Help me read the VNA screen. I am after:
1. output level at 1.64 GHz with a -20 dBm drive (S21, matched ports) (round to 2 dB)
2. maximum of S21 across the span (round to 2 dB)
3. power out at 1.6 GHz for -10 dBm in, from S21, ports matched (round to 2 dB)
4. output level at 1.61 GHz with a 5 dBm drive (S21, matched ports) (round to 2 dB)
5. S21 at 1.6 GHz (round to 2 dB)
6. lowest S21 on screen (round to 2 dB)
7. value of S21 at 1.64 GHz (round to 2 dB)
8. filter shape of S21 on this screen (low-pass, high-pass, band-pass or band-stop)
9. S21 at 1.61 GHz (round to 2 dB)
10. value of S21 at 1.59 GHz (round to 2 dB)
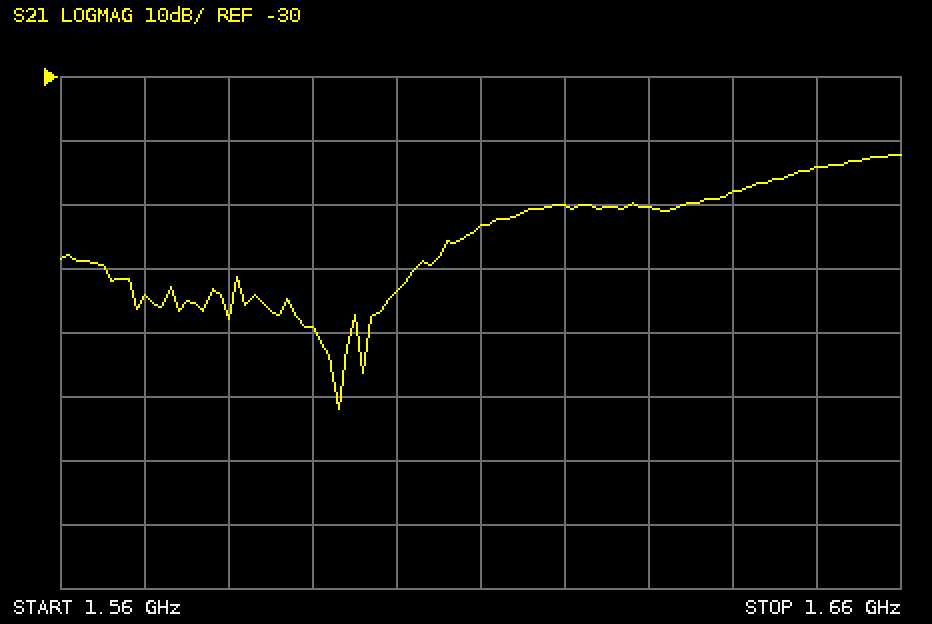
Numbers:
-68 dBm
-42 dB
-74 dBm
-48 dBm
-64 dB
-82 dB
-48 dB
high-pass
-54 dB
-70 dB
